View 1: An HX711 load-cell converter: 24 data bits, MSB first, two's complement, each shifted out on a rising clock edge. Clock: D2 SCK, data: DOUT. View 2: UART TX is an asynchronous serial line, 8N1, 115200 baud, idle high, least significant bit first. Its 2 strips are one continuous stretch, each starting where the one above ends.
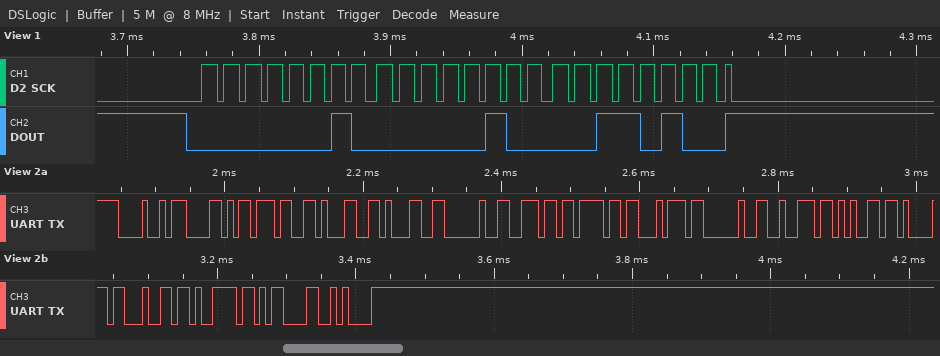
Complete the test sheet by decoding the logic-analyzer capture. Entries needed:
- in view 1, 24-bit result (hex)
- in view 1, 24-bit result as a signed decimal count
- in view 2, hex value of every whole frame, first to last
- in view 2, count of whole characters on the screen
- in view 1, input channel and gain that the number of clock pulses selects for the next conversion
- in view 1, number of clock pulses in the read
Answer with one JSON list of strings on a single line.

["0x020434", "132148", "48 58 37 31 31 20 6E 6F 74 20 72 65 61 64 79 0D 0A", "17", "channel A, gain 128", "25"]
